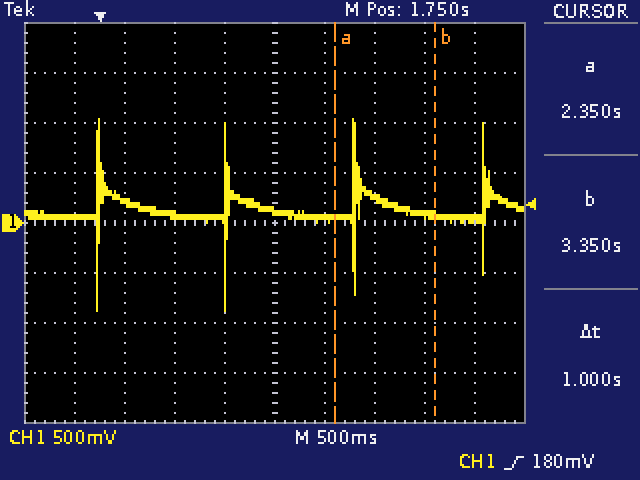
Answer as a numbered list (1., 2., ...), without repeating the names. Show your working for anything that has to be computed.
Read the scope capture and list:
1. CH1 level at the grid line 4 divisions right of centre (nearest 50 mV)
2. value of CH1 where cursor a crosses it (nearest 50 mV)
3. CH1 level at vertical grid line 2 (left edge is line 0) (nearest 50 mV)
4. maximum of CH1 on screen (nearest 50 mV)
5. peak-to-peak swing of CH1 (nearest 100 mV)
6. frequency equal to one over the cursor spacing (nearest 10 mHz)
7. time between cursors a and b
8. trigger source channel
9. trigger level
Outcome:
1. 50 mV
2. 50 mV
3. 200 mV
4. 1.05 V
5. 1.90 V
6. 1 / 1 s ≈ 1.00 Hz
7. 1 s
8. CH1
9. 180 mV
